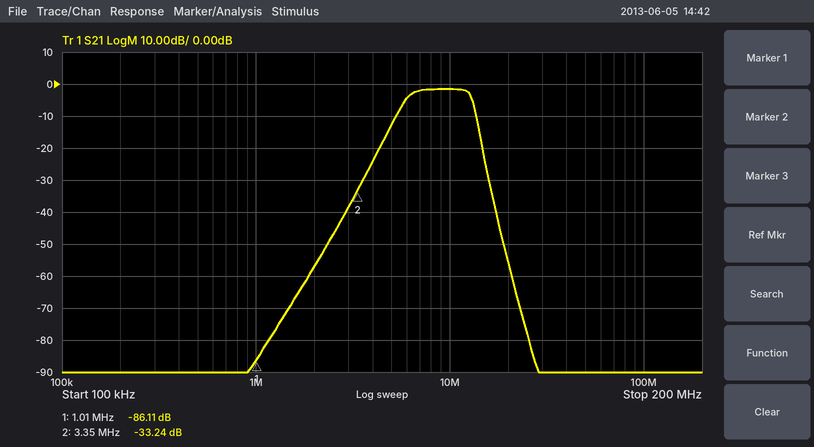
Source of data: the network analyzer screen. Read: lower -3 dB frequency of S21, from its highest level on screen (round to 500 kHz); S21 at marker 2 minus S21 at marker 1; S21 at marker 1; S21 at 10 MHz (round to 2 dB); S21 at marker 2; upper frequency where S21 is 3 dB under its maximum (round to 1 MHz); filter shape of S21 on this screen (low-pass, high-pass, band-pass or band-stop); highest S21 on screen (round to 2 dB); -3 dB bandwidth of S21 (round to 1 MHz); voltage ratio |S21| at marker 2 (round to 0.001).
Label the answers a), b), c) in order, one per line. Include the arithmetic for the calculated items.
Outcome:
a) 6.0 MHz
b) -33.24 − (-86.11) = 52.87 dB
c) -86.11 dB
d) -2 dB
e) -33.24 dB
f) 13 MHz
g) band-pass
h) -2 dB
i) 13 MHz − 6.0 MHz = 7.0 MHz
j) 10^(-33.24/20) ≈ 0.022
